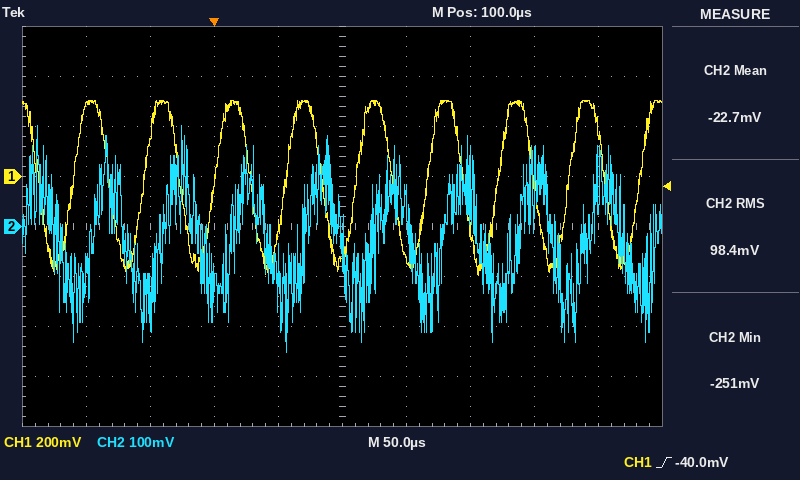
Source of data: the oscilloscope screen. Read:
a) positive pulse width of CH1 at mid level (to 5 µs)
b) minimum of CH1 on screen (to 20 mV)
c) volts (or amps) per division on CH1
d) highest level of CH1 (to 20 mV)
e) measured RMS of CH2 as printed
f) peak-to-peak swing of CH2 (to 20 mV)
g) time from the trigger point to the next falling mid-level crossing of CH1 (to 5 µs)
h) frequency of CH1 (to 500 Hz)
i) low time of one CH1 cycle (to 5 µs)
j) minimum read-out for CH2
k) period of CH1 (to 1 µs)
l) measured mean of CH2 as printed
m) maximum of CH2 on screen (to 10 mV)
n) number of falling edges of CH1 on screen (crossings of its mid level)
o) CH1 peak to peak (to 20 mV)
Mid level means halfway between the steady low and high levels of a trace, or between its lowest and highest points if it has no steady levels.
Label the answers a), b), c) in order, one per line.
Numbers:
a) 30 µs
b) -400 mV
c) 200 mV
d) 300 mV
e) 98.4 mV
f) 460 mV
g) 30 µs
h) 18.0 kHz
i) 25 µs
j) -251 mV
k) 55 µs
l) -22.7 mV
m) 200 mV
n) 9
o) 700 mV
